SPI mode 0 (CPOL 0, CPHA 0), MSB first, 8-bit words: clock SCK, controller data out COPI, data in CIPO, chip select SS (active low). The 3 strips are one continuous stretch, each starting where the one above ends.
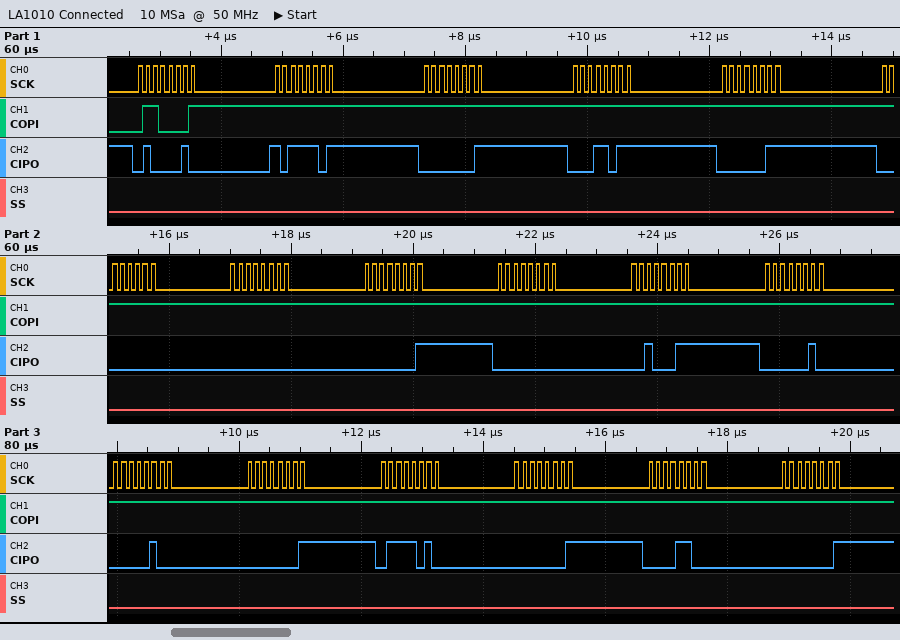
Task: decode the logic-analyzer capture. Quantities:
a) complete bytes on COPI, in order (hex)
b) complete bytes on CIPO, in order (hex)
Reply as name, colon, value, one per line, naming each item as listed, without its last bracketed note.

complete bytes on COPI, in order: 61 FF FF FF FF FF FF FF FF FF FF FF FF FF FF FF FF
complete bytes on CIPO, in order: 42 BD 01 1B 03 00 00 01 00 23 02 04 01 7A 01 0C 01
